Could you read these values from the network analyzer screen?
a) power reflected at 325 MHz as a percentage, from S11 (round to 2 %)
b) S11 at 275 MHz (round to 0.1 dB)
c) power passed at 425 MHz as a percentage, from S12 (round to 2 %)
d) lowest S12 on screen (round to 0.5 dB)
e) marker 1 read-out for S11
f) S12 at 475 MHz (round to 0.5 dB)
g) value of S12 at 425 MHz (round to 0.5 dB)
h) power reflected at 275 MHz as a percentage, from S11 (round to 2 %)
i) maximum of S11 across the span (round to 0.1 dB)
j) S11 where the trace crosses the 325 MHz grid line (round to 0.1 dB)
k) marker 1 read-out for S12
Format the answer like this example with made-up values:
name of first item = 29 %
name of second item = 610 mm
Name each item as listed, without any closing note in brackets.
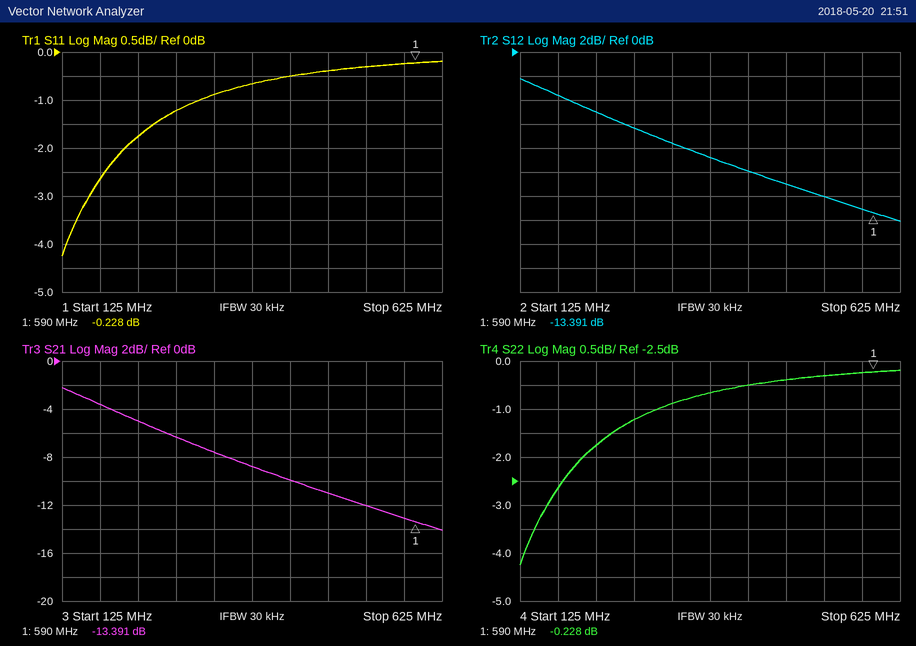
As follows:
power reflected at 325 MHz as a percentage, from S11 = 82 %
S11 at 275 MHz = -1.2 dB
power passed at 425 MHz as a percentage, from S12 = 10 %
lowest S12 on screen = -14.0 dB
marker 1 read-out for S11 = -0.228 dB
S12 at 475 MHz = -11.0 dB
value of S12 at 425 MHz = -10.0 dB
power reflected at 275 MHz as a percentage, from S11 = 76 %
maximum of S11 across the span = -0.2 dB
S11 where the trace crosses the 325 MHz grid line = -0.9 dB
marker 1 read-out for S12 = -13.391 dB
